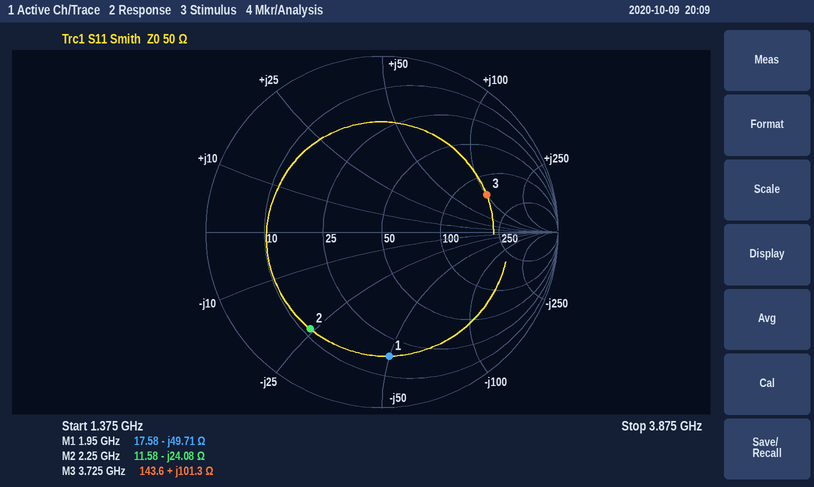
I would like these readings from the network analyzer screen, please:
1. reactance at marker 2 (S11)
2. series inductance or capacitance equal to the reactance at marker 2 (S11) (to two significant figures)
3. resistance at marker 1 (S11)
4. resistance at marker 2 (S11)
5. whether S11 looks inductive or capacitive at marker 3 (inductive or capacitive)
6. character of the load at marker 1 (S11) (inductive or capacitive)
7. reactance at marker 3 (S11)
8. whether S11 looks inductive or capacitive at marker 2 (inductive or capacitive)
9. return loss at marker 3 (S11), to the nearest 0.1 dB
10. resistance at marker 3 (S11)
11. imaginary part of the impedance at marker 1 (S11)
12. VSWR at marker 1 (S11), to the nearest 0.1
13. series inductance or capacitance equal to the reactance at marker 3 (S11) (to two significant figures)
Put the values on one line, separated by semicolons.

-24.08 Ω; 2.9 pF; 17.58 Ω; 11.58 Ω; inductive; capacitive; +101.3 Ω; capacitive; 4.0 dB; 143.6 Ω; -49.71 Ω; 5.8; 4.3 nH
